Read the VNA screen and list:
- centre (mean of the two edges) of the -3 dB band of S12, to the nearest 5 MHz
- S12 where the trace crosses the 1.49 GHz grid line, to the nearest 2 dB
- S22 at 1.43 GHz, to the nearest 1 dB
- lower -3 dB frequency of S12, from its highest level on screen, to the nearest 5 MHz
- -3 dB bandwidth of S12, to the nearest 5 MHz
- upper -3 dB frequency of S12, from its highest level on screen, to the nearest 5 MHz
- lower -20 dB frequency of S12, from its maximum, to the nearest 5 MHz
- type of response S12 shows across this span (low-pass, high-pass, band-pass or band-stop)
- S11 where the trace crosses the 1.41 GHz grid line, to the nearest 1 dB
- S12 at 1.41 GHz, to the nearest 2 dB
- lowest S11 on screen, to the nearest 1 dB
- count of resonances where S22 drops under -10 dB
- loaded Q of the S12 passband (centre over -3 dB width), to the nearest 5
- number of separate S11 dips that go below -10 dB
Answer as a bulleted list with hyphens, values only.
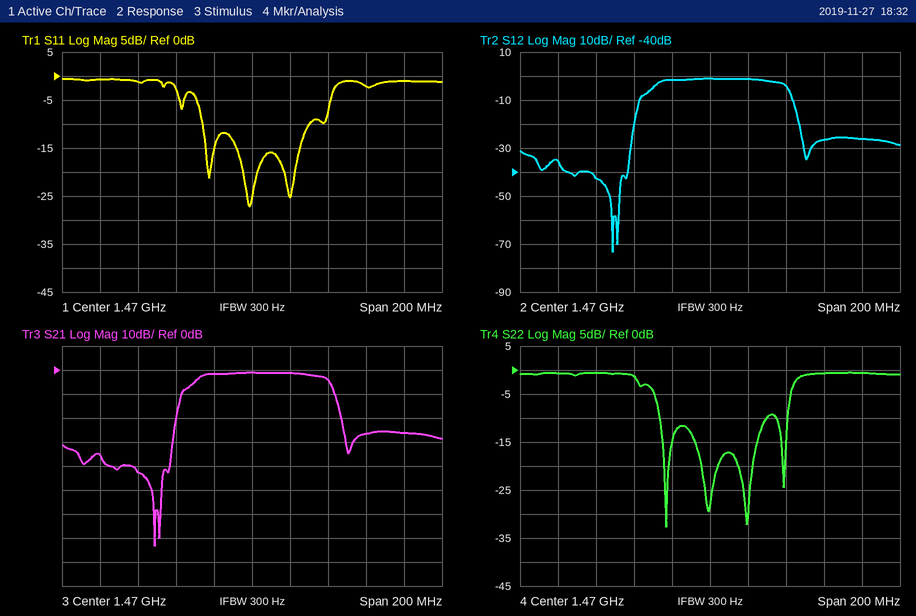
- 1.475 GHz
- -2 dB
- -1 dB
- 1.440 GHz
- 70 MHz
- 1.510 GHz
- 1.430 GHz
- band-pass
- -1 dB
- -42 dB
- -27 dB
- 4
- 20
- 3
